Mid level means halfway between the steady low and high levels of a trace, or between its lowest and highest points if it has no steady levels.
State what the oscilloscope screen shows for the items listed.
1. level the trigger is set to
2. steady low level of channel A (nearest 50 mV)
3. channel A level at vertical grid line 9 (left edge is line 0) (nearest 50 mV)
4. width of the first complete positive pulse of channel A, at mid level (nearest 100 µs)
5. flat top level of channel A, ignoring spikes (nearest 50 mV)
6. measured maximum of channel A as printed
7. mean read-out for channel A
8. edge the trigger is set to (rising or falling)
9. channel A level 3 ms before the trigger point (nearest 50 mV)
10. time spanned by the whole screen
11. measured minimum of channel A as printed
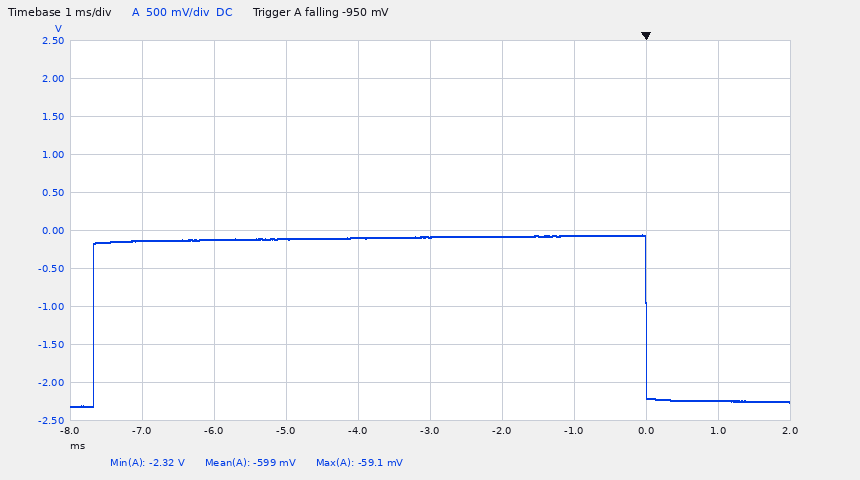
-950 mV
-2.25 V
-2.25 V
7.7 ms
-100 mV
-59.1 mV
-599 mV
falling
-100 mV
10 ms
-2.32 V
